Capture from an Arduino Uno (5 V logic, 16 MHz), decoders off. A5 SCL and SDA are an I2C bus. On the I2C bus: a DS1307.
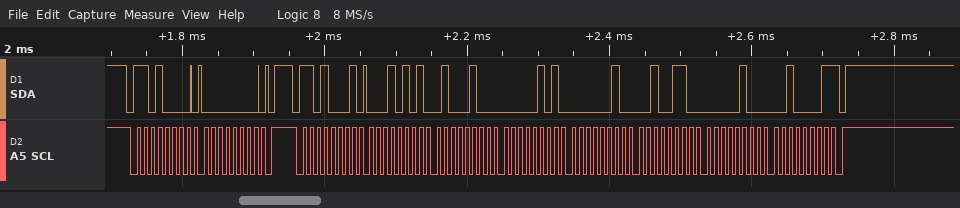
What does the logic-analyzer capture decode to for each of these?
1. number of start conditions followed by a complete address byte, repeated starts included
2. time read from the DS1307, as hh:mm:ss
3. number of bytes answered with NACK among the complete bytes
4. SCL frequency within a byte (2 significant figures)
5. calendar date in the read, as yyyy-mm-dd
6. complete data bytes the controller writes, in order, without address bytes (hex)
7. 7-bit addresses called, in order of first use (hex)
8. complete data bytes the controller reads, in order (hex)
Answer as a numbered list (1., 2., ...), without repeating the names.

1. 2
2. 05:44:15
3. 1
4. 100 kHz
5. 2021-04-26
6. 00
7. 0x68
8. 15 44 05 02 26 04 21
